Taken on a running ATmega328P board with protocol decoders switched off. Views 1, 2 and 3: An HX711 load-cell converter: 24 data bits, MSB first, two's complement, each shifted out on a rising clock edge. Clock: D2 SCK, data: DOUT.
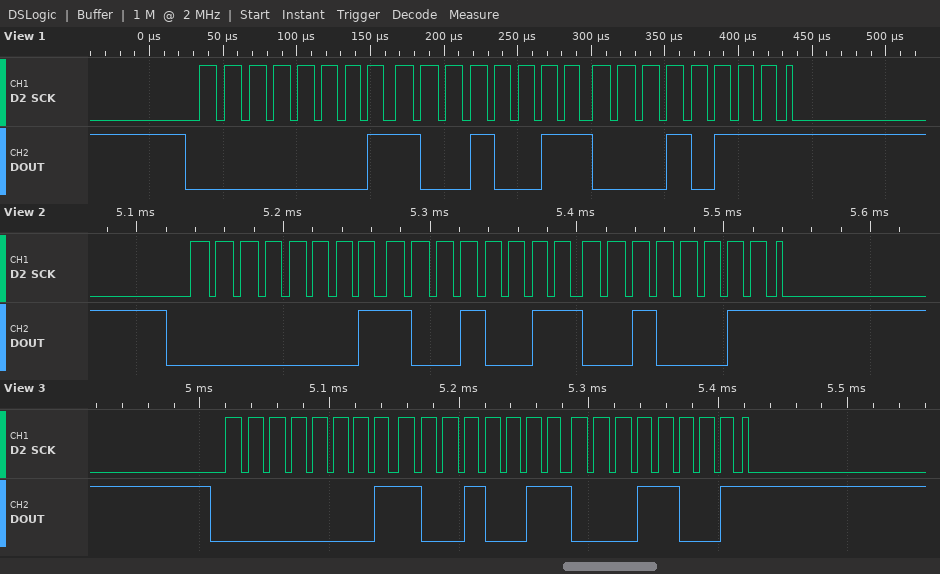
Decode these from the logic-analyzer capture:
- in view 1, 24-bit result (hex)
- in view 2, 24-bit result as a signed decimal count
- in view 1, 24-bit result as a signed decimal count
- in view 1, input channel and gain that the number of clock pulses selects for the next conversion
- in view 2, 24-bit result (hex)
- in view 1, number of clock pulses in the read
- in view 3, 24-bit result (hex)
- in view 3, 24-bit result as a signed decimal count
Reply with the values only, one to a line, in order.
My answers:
0x019317
103203
103191
channel A, gain 128
0x019323
25
0x019319
103193
